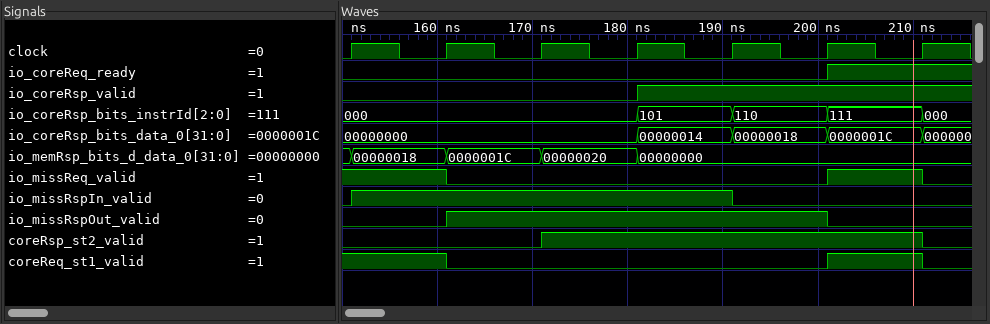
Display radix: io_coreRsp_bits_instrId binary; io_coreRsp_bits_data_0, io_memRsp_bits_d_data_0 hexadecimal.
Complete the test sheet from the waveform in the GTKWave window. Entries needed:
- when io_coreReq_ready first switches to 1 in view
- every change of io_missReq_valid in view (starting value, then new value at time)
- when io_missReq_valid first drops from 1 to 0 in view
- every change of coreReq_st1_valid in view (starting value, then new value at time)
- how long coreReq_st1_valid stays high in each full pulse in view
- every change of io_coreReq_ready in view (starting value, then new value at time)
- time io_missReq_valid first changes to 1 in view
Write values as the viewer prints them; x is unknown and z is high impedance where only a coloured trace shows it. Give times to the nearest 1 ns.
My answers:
201 ns
1, 0 at 161 ns, 1 at 201 ns, 0 at 211 ns
161 ns
1, 0 at 161 ns, 1 at 201 ns, 0 at 211 ns
10 ns
0, 1 at 201 ns
201 ns
